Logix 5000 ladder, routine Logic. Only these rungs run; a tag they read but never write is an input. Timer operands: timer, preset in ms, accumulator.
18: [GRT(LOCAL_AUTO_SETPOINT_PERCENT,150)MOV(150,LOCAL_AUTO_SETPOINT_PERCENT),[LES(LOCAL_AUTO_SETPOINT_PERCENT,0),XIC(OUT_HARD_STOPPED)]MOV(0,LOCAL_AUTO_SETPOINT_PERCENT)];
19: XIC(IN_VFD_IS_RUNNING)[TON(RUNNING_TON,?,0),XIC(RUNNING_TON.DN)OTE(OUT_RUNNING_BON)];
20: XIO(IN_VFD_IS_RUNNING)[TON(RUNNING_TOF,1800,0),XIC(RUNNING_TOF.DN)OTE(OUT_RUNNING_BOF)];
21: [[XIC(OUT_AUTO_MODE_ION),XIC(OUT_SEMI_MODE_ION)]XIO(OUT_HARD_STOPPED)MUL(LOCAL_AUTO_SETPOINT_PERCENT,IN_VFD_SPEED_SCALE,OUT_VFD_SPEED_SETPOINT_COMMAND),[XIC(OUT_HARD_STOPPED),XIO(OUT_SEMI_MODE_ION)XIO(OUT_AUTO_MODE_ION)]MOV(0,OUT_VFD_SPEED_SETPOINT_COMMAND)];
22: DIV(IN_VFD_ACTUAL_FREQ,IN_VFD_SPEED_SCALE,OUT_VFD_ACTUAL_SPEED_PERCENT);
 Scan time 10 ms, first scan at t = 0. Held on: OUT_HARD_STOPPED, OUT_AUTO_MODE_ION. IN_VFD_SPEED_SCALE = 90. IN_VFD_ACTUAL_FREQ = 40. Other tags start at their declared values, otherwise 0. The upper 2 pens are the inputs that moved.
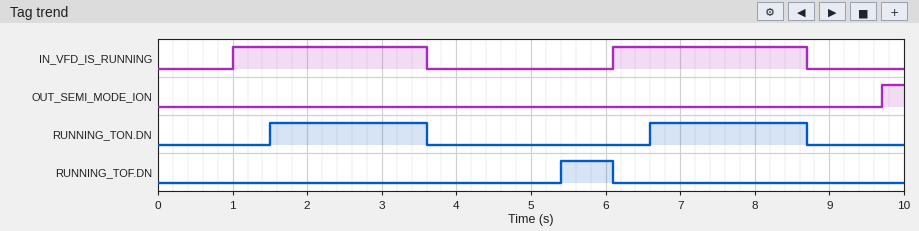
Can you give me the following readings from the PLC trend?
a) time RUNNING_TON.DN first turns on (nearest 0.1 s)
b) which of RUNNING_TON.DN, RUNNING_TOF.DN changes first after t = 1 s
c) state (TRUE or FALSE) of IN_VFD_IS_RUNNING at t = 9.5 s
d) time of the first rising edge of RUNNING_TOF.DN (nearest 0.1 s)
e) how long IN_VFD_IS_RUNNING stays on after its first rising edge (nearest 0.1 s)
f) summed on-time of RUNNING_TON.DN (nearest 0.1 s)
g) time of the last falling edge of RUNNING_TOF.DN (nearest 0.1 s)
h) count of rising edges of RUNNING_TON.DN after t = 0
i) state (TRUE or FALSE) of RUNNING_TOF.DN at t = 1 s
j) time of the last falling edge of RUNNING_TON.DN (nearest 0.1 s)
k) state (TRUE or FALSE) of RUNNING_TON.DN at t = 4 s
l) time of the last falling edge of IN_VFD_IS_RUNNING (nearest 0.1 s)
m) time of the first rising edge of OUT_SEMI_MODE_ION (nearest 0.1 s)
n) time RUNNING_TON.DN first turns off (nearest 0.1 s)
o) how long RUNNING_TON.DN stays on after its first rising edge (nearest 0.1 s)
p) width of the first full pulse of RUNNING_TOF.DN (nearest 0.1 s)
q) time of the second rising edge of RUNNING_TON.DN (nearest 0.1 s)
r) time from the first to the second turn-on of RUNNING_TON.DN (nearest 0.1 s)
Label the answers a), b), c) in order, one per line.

a) 1.5 s
b) RUNNING_TON.DN
c) FALSE
d) 5.4 s
e) 2.6 s
f) 4.2 s
g) 6.1 s
h) 2
i) FALSE
j) 8.7 s
k) FALSE
l) 8.7 s
m) 9.7 s
n) 3.6 s
o) 2.1 s
p) 0.7 s
q) 6.6 s
r) 5.1 s
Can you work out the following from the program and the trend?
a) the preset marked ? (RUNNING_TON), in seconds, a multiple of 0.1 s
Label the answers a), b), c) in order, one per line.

a) 0.5 s
